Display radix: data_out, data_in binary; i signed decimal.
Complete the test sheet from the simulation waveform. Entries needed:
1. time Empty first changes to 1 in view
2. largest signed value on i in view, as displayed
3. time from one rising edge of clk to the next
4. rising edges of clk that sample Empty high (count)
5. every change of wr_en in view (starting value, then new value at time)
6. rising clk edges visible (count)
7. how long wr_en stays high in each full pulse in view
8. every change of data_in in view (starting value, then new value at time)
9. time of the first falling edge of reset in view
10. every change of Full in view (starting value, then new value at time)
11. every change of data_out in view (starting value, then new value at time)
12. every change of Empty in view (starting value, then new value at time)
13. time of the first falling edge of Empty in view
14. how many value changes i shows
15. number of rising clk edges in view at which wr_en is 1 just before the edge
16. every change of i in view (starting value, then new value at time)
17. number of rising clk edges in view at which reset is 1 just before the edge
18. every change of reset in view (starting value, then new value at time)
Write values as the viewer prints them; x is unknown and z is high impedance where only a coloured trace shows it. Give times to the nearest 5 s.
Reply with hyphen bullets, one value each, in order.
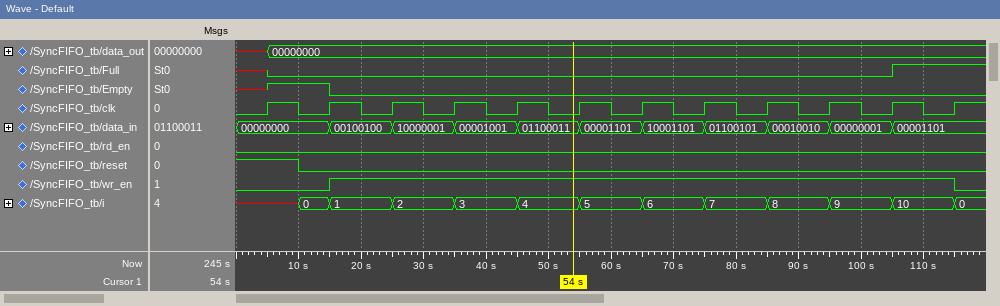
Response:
- 5 s
- 10
- 10 s
- 1
- 0, 1 at 15 s, 0 at 115 s
- 12
- 100 s
- 00000000, 00100100 at 15 s, 10000001 at 25 s, 00001001 at 35 s, 01100011 at 45 s, 00001101 at 55 s, 10001101 at 65 s, 01100101 at 75 s, 00010010 at 85 s, 00000001 at 95 s, 00001101 at 105 s
- 10 s
- x, 0 at 5 s, 1 at 105 s
- x, 00000000 at 5 s
- x, 1 at 5 s, 0 at 15 s
- 15 s
- 12
- 10
- x, 0 at 10 s, 1 at 15 s, 2 at 25 s, 3 at 35 s, 4 at 45 s, 5 at 55 s, 6 at 65 s, 7 at 75 s, 8 at 85 s, 9 at 95 s, 10 at 105 s, 0 at 115 s
- 1
- 1, 0 at 10 s
